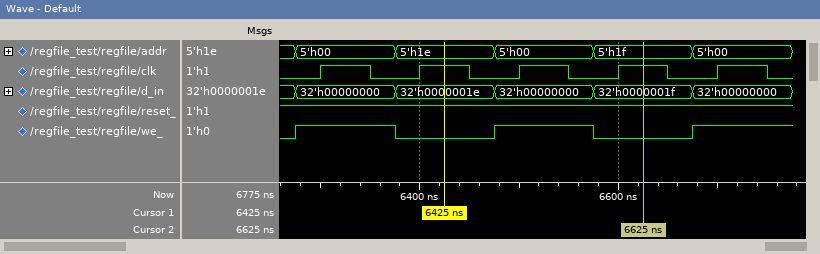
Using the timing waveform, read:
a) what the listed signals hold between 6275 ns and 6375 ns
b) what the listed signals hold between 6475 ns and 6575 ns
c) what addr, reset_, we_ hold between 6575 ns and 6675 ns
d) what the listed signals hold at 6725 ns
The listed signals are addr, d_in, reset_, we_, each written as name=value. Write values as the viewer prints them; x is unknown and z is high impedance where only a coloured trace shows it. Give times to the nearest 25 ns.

addr=5'h00, d_in=32'h00000000, reset_=1, we_=1
addr=5'h00, d_in=32'h00000000, reset_=1, we_=1
addr=5'h1f, reset_=1, we_=0
addr=5'h00, d_in=32'h00000000, reset_=1, we_=1
